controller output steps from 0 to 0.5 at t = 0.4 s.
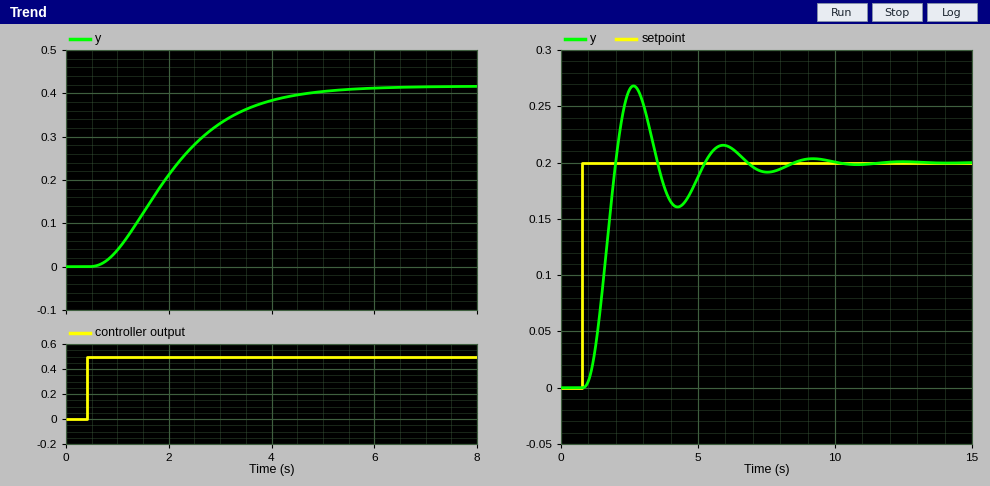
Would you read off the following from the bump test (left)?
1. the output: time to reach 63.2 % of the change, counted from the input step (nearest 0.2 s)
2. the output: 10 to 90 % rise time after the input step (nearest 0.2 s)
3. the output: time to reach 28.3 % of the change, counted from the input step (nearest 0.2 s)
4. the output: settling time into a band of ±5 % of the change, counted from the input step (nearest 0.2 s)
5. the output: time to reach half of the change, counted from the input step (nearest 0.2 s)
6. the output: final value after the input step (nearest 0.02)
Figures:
2.0 s
2.8 s
1.0 s
4.0 s
1.6 s
0.42
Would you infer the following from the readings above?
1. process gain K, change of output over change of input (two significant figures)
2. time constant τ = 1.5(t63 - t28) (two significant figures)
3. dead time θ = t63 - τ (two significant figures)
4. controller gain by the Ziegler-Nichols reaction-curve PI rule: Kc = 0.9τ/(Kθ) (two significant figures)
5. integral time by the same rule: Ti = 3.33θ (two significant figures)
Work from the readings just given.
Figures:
0.84
1.5 s
0.50 s
3.2
1.7 s
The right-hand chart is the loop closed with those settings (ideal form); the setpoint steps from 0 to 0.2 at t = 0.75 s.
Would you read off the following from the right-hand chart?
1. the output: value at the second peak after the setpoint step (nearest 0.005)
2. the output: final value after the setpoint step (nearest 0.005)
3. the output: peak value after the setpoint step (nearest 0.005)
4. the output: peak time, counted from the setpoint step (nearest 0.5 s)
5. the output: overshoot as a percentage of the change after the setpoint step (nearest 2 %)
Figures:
0.215
0.200
0.270
2.0 s
34 %
